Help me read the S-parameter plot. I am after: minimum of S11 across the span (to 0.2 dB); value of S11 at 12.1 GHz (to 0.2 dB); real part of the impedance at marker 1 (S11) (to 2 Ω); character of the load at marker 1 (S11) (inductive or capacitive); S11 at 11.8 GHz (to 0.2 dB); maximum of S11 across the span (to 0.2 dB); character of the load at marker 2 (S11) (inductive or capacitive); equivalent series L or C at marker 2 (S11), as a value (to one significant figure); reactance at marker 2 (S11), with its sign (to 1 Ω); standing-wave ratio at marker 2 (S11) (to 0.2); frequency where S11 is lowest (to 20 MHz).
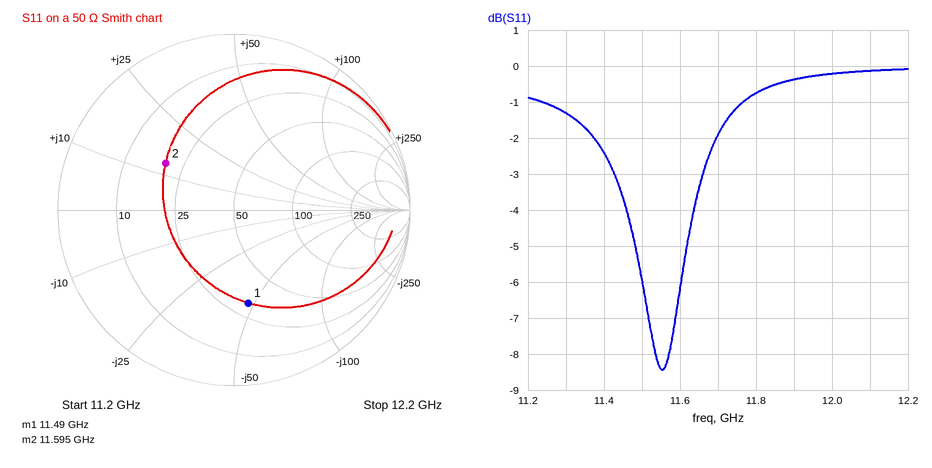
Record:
-8.4 dB
-0.2 dB
32 Ω
capacitive
-0.8 dB
0.0 dB
inductive
200 pH
+13 Ω
2.8
11.56 GHz
